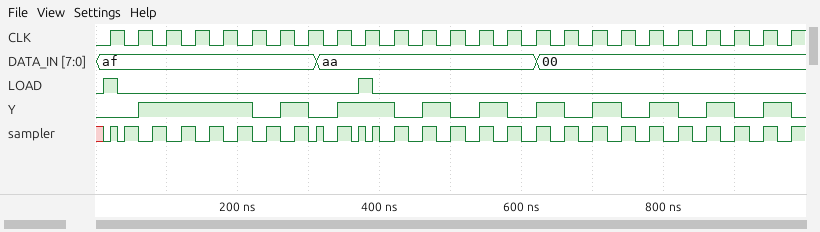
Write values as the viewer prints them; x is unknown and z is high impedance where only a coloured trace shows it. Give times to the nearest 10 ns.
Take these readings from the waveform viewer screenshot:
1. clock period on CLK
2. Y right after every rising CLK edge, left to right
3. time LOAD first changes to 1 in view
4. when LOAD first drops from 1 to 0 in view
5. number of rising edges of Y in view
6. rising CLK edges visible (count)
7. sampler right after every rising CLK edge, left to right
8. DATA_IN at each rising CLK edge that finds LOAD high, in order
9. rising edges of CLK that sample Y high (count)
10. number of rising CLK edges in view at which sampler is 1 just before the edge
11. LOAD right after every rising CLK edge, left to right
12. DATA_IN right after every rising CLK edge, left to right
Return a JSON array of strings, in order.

["40 ns", "0 1 1 1 1 0 1 0 1 1 0 1 0 1 0 1 0 1 0 1 0 1 0 1 0", "10 ns", "30 ns", "10", "25", "1 0 0 0 0 0 0 0 1 0 1 1 1 1 1 1 1 1 1 1 1 1 1 1 1", "af, aa", "14", "8", "1 0 0 0 0 0 0 0 0 1 0 0 0 0 0 0 0 0 0 0 0 0 0 0 0", "af, af, af, af, af, af, af, af, aa, aa, aa, aa, aa, aa, aa, 00, 00, 00, 00, 00, 00, 00, 00, 00, 00"]
